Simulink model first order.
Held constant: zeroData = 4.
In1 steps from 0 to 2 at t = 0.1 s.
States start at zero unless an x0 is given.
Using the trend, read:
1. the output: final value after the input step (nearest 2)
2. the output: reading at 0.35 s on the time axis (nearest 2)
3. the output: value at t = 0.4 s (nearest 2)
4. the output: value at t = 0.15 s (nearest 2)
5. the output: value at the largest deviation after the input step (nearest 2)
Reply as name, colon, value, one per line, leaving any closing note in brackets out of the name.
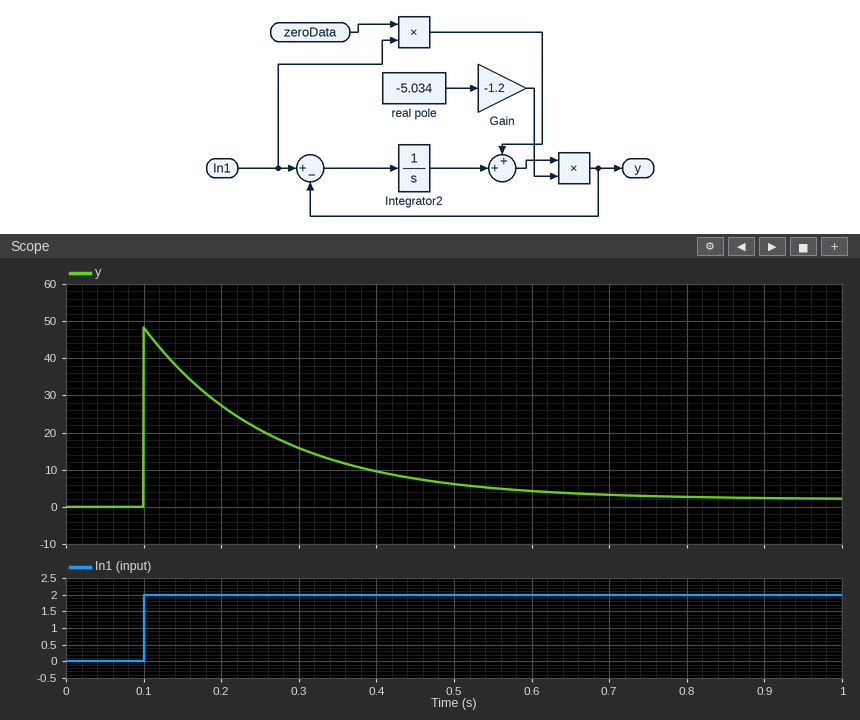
the output: final value after the input step: 2
the output: reading at 0.35 s on the time axis: 12
the output: value at t = 0.4 s: 10
the output: value at t = 0.15 s: 36
the output: value at the largest deviation after the input step: 48
